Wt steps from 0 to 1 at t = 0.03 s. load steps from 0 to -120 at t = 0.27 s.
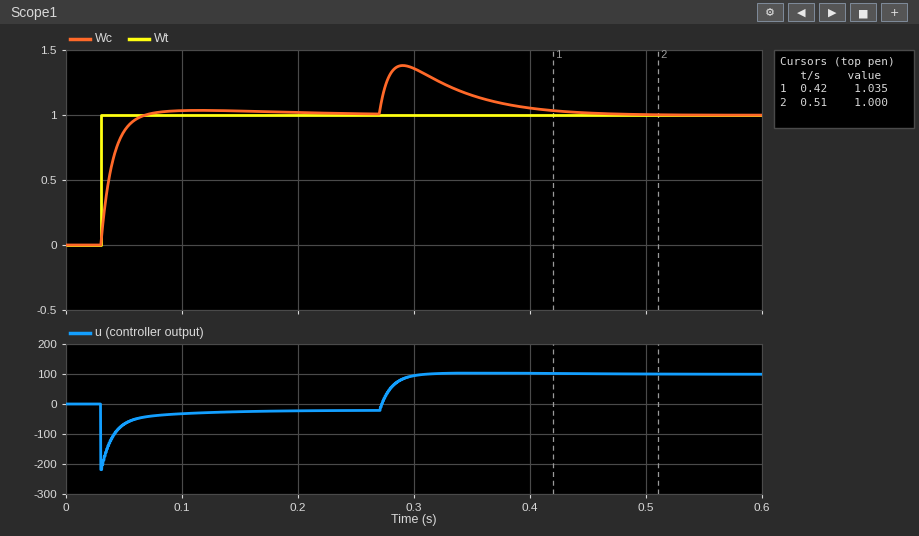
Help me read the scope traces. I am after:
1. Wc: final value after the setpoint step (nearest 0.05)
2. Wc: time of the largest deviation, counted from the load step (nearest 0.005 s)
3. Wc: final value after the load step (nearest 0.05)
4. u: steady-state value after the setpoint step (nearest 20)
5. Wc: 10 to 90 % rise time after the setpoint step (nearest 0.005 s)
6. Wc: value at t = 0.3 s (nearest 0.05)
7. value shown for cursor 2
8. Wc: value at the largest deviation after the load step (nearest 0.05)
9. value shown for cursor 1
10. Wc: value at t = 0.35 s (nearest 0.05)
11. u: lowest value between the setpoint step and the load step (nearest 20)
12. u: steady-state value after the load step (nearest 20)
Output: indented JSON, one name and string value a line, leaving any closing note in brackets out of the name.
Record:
{
  "Wc: final value after the setpoint step": "1.00",
  "Wc: time of the largest deviation, counted from the load step": "0.020 s",
  "Wc: final value after the load step": "1.00",
  "u: steady-state value after the setpoint step": "-20",
  "Wc: 10 to 90 % rise time after the setpoint step": "0.020 s",
  "Wc: value at t = 0.3 s": "1.35",
  "value shown for cursor 2": "1.000",
  "Wc: value at the largest deviation after the load step": "1.40",
  "value shown for cursor 1": "1.035",
  "Wc: value at t = 0.35 s": "1.15",
  "u: lowest value between the setpoint step and the load step": "-220",
  "u: steady-state value after the load step": "100"
}
